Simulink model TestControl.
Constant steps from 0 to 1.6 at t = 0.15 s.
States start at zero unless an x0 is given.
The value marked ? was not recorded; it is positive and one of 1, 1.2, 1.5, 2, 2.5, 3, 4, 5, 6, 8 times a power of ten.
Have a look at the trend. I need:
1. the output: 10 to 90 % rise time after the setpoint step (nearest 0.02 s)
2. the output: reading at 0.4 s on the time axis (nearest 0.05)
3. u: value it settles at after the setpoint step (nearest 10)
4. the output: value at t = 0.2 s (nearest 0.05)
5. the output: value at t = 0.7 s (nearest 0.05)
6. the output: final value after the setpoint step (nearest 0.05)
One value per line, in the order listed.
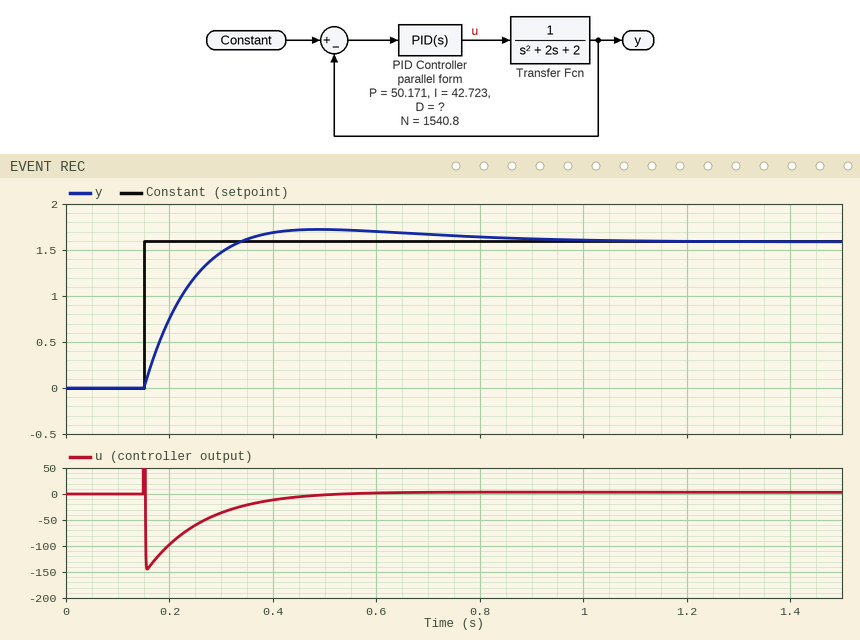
0.14 s
1.70
0
0.75
1.65
1.60
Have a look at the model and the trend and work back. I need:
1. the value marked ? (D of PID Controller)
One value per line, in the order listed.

12
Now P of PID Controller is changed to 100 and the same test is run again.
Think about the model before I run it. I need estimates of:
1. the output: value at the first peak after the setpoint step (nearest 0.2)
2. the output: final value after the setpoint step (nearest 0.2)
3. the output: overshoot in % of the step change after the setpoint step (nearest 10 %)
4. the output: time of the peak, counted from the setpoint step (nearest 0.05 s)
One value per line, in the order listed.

1.8
1.6
20 %
0.25 s
